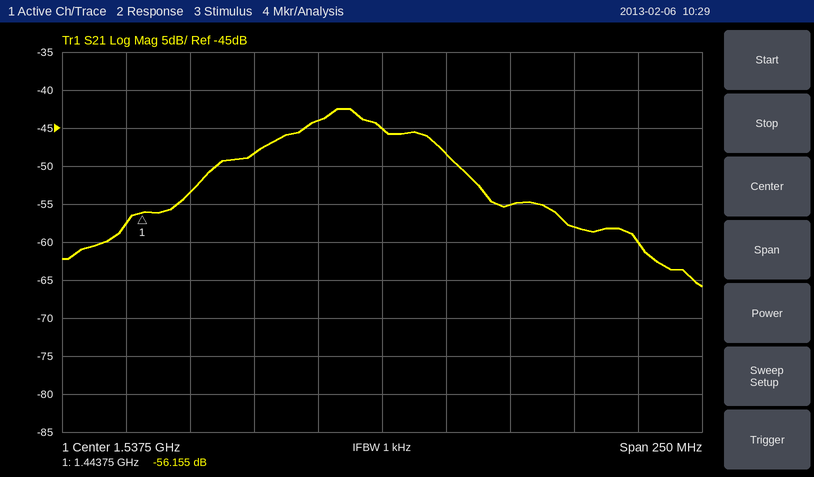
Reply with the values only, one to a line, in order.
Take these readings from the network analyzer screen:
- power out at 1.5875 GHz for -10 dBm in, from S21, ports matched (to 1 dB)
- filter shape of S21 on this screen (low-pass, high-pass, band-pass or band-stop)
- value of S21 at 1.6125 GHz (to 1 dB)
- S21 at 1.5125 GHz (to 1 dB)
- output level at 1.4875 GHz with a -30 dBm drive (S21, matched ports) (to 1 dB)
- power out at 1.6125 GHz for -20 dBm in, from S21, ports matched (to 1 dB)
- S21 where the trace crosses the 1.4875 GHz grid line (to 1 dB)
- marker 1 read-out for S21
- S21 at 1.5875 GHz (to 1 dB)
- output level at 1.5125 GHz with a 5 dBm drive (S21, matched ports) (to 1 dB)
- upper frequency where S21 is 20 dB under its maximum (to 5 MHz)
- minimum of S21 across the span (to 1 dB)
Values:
-65 dBm
band-pass
-58 dB
-44 dB
-78 dBm
-78 dBm
-48 dB
-56.155 dB
-55 dB
-39 dBm
1.645 GHz
-66 dB
